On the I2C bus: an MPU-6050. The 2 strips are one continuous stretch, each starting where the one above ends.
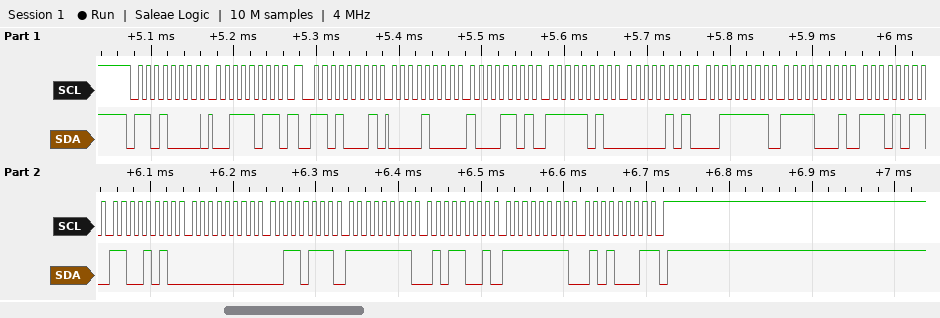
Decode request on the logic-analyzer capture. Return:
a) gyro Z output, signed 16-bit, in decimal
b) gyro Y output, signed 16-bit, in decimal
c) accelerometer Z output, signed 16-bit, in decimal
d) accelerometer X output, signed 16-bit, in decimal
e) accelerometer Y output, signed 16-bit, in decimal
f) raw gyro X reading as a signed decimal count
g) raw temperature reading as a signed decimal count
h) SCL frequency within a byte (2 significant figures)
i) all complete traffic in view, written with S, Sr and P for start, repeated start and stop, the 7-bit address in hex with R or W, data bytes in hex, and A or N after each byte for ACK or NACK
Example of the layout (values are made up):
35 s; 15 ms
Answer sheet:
-175; -167; 16369; 2189; -1531; 55; -5174; 100 kHz; S 68W A 3B A Sr 68R A 08 A 8D A FA A 05 A 3F A F1 A EB A CA A 00 A 37 A FF A 59 A FF A 51 N P
